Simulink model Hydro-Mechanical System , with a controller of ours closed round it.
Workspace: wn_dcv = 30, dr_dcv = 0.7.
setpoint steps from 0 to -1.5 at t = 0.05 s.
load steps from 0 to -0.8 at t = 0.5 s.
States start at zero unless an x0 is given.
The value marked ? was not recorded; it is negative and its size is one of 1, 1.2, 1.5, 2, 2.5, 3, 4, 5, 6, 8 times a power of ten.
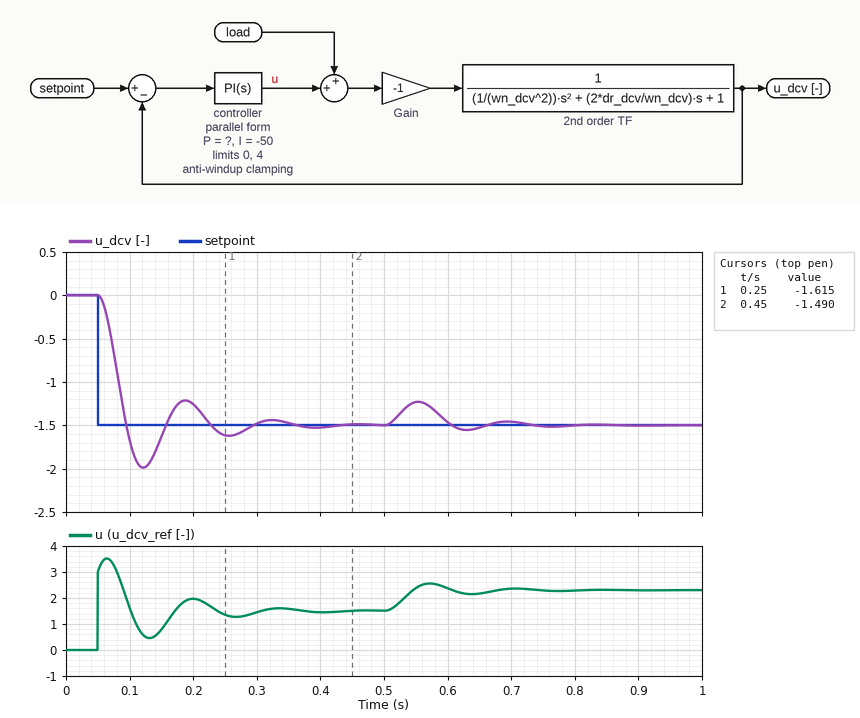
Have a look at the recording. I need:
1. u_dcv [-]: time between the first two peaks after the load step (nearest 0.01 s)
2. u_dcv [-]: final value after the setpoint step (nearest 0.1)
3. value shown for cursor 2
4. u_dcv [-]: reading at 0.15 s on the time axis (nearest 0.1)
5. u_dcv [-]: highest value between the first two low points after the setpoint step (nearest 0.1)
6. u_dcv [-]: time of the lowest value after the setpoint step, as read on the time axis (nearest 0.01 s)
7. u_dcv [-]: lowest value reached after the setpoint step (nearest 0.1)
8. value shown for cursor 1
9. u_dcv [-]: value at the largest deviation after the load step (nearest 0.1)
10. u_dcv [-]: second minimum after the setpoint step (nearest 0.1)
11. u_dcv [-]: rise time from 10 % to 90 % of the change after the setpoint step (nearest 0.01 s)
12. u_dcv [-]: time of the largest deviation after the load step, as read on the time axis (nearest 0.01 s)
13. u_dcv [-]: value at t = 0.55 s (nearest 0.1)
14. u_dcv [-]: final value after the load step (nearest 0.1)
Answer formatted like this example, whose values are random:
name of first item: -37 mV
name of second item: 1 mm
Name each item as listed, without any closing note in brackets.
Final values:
u_dcv [-]: time between the first two peaks after the load step: 0.14 s
u_dcv [-]: final value after the setpoint step: -1.5
value shown for cursor 2: -1.490
u_dcv [-]: reading at 0.15 s on the time axis: -1.6
u_dcv [-]: highest value between the first two low points after the setpoint step: -1.2
u_dcv [-]: time of the lowest value after the setpoint step, as read on the time axis: 0.12 s
u_dcv [-]: lowest value reached after the setpoint step: -2.0
value shown for cursor 1: -1.615
u_dcv [-]: value at the largest deviation after the load step: -1.2
u_dcv [-]: second minimum after the setpoint step: -1.6
u_dcv [-]: rise time from 10 % to 90 % of the change after the setpoint step: 0.03 s
u_dcv [-]: time of the largest deviation after the load step, as read on the time axis: 0.55 s
u_dcv [-]: value at t = 0.55 s: -1.2
u_dcv [-]: final value after the load step: -1.5
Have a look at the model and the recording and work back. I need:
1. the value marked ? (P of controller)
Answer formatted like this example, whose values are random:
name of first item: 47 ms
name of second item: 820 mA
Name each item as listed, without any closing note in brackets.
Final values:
the value marked ?: -2
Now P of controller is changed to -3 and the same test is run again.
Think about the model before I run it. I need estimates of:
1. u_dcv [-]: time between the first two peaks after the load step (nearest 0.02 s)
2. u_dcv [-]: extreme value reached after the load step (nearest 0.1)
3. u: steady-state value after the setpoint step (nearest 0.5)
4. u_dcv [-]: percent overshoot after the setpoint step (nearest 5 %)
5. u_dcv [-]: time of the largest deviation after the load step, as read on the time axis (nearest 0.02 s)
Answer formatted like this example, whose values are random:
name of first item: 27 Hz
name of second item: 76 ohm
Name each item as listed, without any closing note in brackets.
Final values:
u_dcv [-]: time between the first two peaks after the load step: 0.12 s
u_dcv [-]: extreme value reached after the load step: -1.3
u: steady-state value after the setpoint step: 1.5
u_dcv [-]: percent overshoot after the setpoint step: 15 %
u_dcv [-]: time of the largest deviation after the load step, as read on the time axis: 0.54 s
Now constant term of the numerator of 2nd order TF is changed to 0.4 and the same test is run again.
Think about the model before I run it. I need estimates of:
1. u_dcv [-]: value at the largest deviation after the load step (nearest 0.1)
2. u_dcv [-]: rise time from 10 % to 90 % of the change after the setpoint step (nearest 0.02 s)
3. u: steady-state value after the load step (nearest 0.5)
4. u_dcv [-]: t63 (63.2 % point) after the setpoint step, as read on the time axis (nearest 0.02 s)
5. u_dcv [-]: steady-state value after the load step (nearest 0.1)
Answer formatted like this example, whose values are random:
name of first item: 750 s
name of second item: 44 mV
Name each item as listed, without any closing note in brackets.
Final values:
u_dcv [-]: value at the largest deviation after the load step: -1.3
u_dcv [-]: rise time from 10 % to 90 % of the change after the setpoint step: 0.06 s
u: steady-state value after the load step: 4.0
u_dcv [-]: t63 (63.2 % point) after the setpoint step, as read on the time axis: 0.10 s
u_dcv [-]: steady-state value after the load step: -1.3
